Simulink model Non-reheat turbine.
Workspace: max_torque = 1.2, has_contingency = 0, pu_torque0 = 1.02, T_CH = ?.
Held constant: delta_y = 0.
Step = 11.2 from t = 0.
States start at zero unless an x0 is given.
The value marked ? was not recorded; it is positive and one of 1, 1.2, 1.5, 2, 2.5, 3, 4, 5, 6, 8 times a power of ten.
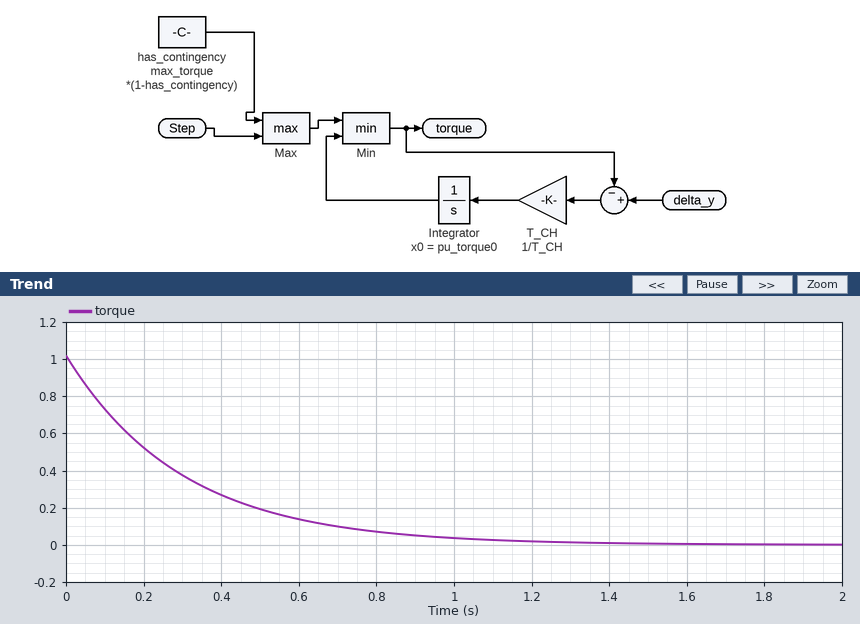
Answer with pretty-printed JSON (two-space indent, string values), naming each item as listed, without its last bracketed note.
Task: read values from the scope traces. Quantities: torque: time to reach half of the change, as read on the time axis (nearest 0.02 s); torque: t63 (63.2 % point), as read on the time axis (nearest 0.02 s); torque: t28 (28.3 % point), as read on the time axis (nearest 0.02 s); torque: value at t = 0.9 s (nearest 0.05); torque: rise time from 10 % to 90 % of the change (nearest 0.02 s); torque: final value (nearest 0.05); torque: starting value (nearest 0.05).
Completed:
{
  "torque: time to reach half of the change, as read on the time axis": "0.20 s",
  "torque: t63 (63.2 % point), as read on the time axis": "0.30 s",
  "torque: t28 (28.3 % point), as read on the time axis": "0.10 s",
  "torque: value at t = 0.9 s": "0.05",
  "torque: rise time from 10 % to 90 % of the change": "0.66 s",
  "torque: final value": "0.00",
  "torque: starting value": "1.00"
}
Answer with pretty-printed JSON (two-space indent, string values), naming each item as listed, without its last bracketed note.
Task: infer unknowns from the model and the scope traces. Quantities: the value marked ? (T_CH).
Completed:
{
  "the value marked ?": "0.3"
}
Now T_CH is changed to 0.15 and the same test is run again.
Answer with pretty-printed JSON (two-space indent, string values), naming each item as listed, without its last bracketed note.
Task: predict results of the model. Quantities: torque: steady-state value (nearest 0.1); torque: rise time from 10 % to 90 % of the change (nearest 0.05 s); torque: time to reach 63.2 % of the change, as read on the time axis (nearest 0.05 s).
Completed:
{
  "torque: steady-state value": "0.0",
  "torque: rise time from 10 % to 90 % of the change": "0.35 s",
  "torque: time to reach 63.2 % of the change, as read on the time axis": "0.15 s"
}
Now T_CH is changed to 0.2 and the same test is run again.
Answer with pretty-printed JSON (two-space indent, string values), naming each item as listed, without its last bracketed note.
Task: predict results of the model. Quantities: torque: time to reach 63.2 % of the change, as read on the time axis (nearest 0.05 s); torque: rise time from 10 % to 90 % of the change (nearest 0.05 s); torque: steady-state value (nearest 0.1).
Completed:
{
  "torque: time to reach 63.2 % of the change, as read on the time axis": "0.20 s",
  "torque: rise time from 10 % to 90 % of the change": "0.45 s",
  "torque: steady-state value": "0.0"
}
